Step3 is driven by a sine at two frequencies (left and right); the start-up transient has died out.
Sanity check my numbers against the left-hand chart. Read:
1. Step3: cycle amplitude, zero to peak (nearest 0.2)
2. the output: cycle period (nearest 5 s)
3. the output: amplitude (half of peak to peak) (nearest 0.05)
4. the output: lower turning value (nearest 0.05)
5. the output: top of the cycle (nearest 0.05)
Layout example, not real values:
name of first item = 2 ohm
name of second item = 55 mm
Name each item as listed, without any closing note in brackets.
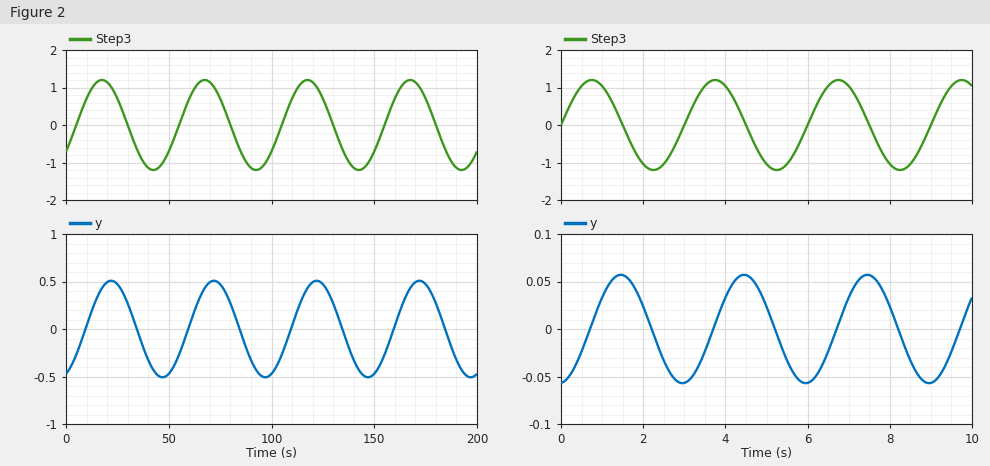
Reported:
Step3: cycle amplitude, zero to peak = 1.2
the output: cycle period = 50 s
the output: amplitude (half of peak to peak) = 0.50
the output: lower turning value = -0.50
the output: top of the cycle = 0.50
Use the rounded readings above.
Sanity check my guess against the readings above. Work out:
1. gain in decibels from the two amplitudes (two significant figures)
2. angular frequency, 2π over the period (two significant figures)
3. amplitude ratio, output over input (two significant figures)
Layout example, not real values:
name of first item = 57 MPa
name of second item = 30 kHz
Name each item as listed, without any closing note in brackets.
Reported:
gain in decibels from the two amplitudes = -7.6 dB
angular frequency, 2π over the period = 0.13 rad/s
amplitude ratio, output over input = 0.42
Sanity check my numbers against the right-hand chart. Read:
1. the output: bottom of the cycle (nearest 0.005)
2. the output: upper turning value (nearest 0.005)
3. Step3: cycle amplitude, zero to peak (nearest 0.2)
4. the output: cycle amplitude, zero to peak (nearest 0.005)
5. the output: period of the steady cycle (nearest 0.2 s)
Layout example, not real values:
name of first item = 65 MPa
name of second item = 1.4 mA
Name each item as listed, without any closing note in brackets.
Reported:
the output: bottom of the cycle = -0.055
the output: upper turning value = 0.055
Step3: cycle amplitude, zero to peak = 1.2
the output: cycle amplitude, zero to peak = 0.055
the output: period of the steady cycle = 3.0 s
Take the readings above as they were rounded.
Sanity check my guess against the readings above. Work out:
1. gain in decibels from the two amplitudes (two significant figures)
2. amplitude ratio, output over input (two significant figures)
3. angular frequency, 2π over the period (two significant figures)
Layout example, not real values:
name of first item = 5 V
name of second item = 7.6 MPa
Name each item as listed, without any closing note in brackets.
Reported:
gain in decibels from the two amplitudes = -27 dB
amplitude ratio, output over input = 0.046
angular frequency, 2π over the period = 2.1 rad/s
